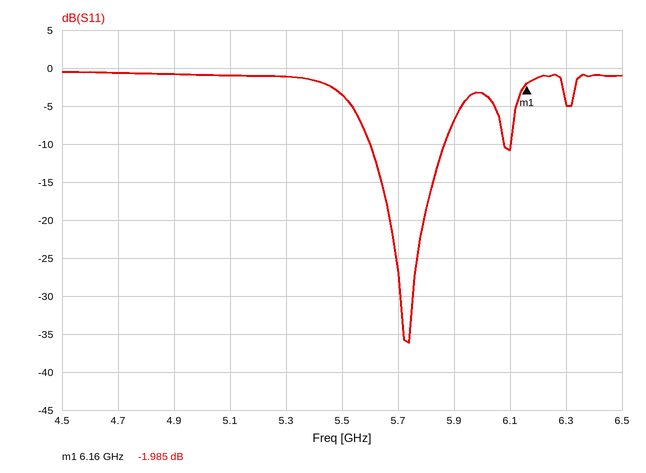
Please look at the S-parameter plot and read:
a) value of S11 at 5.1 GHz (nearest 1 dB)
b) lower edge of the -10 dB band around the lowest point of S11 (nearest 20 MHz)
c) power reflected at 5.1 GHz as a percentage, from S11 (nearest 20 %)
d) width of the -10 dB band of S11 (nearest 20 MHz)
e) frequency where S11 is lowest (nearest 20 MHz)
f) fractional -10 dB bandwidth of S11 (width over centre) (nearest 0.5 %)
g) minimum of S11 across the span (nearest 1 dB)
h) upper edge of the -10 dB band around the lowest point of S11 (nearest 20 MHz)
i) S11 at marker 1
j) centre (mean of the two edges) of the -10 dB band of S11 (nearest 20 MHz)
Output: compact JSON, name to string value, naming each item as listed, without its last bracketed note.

{"value of S11 at 5.1 GHz": "-1 dB", "lower edge of the -10 dB band around the lowest point of S11": "5.60 GHz", "power reflected at 5.1 GHz as a percentage, from S11": "80 %", "width of the -10 dB band of S11": "260 MHz", "frequency where S11 is lowest": "5.74 GHz", "fractional -10 dB bandwidth of S11 (width over centre)": "4.5 %", "minimum of S11 across the span": "-36 dB", "upper edge of the -10 dB band around the lowest point of S11": "5.86 GHz", "S11 at marker 1": "-1.985 dB", "centre (mean of the two edges) of the -10 dB band of S11": "5.74 GHz"}
